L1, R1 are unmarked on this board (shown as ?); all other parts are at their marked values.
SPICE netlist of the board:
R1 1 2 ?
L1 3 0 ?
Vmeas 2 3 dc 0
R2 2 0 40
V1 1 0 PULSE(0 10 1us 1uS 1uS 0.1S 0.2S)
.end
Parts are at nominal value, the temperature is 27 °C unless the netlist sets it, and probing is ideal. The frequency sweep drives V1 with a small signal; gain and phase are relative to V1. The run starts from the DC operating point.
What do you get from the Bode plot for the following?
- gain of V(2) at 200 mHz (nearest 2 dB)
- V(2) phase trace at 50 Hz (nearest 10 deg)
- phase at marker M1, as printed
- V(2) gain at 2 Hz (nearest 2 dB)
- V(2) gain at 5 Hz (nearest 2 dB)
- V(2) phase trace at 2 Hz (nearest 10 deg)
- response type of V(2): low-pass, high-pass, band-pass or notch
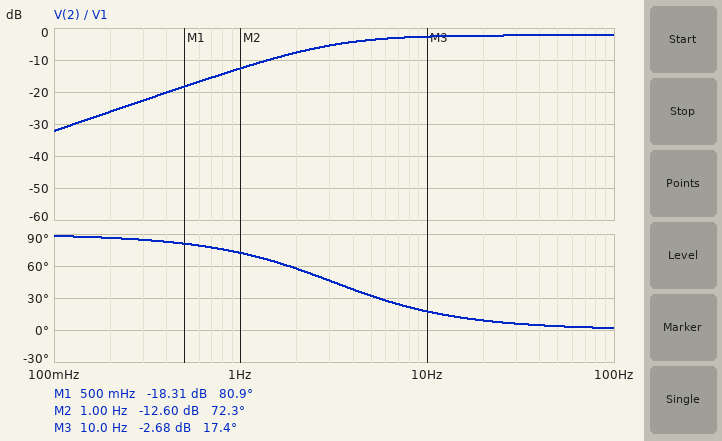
-26 dB
0 deg
80.9 deg
-8 dB
-4 dB
60 deg
high-pass
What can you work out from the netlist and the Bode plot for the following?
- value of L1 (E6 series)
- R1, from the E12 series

470 mH
12 Ω
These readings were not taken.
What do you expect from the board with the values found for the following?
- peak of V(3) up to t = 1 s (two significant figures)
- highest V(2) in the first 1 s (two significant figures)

7.7 V
7.7 V
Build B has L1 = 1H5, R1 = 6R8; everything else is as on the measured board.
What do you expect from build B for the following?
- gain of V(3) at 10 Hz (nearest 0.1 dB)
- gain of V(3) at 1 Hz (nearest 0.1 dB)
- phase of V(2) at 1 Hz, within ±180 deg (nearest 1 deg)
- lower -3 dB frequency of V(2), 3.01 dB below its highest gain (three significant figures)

-1.4 dB
-2.8 dB
32 deg
617 mHz
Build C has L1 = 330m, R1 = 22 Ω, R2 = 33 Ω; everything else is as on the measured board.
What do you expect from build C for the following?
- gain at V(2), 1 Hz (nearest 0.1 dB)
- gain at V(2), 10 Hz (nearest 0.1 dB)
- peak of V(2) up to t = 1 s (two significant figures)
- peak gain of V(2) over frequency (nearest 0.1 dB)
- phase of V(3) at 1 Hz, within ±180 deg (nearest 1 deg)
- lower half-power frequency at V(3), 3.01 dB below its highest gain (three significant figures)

-20.6 dB
-5.9 dB
6.0 V
-4.4 dB
81 deg
6.37 Hz
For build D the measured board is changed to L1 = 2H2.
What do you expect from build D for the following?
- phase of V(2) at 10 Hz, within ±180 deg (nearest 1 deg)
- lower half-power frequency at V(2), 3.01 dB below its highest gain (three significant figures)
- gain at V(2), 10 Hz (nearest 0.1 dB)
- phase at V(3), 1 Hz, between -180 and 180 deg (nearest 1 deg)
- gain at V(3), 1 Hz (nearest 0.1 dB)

4 deg
668 mHz
-2.3 dB
34 deg
-3.9 dB
